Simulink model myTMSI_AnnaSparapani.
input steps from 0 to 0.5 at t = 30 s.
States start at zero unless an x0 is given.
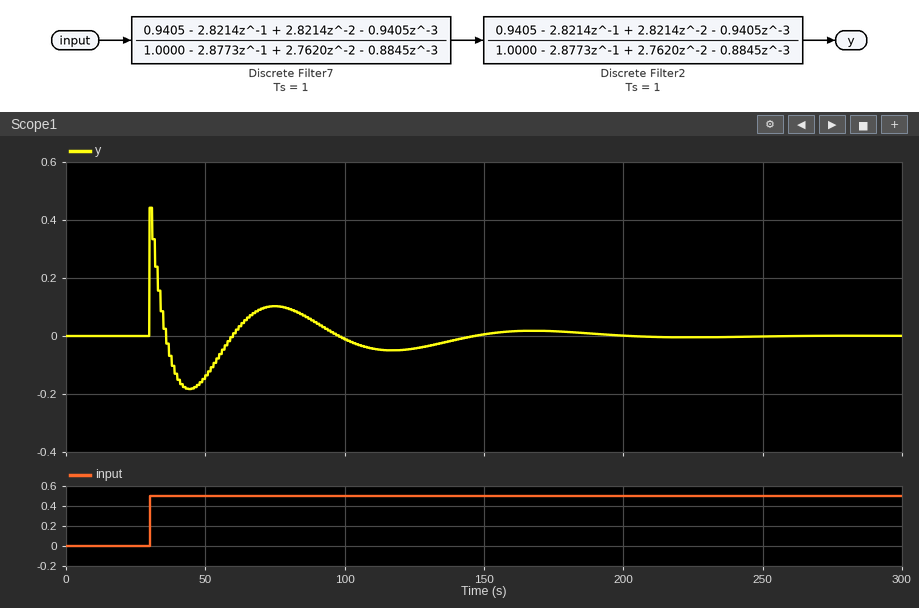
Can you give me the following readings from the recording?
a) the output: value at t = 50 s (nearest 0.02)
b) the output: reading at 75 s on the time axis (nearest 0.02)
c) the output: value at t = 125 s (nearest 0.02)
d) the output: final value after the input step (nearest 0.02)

-0.14
0.10
-0.04
0.00
